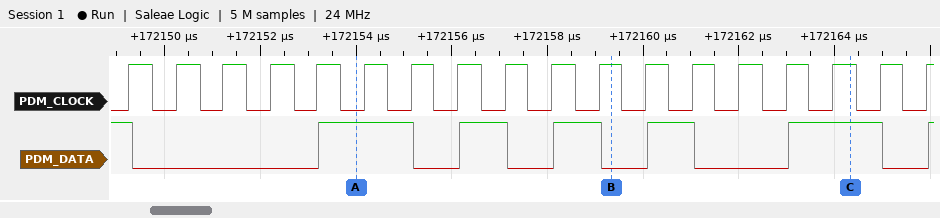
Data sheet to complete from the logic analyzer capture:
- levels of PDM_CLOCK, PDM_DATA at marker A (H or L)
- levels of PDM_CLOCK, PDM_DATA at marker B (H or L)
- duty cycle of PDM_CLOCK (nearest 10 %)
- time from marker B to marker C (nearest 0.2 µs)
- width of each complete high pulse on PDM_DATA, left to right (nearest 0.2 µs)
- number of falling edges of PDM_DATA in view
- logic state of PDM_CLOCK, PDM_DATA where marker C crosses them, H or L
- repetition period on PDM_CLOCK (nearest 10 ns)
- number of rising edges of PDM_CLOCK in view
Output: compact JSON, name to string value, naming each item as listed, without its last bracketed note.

{"levels of PDM_CLOCK, PDM_DATA at marker A": "PDM_CLOCK=L, PDM_DATA=H", "levels of PDM_CLOCK, PDM_DATA at marker B": "PDM_CLOCK=H, PDM_DATA=L", "duty cycle of PDM_CLOCK": "50 %", "time from marker B to marker C": "5 µs", "width of each complete high pulse on PDM_DATA, left to right": "2 µs, 1 µs, 1 µs, 1 µs, 2 µs", "number of falling edges of PDM_DATA in view": "6", "logic state of PDM_CLOCK, PDM_DATA where marker C crosses them, H or L": "PDM_CLOCK=H, PDM_DATA=H", "repetition period on PDM_CLOCK": "980 ns", "number of rising edges of PDM_CLOCK in view": "18"}
